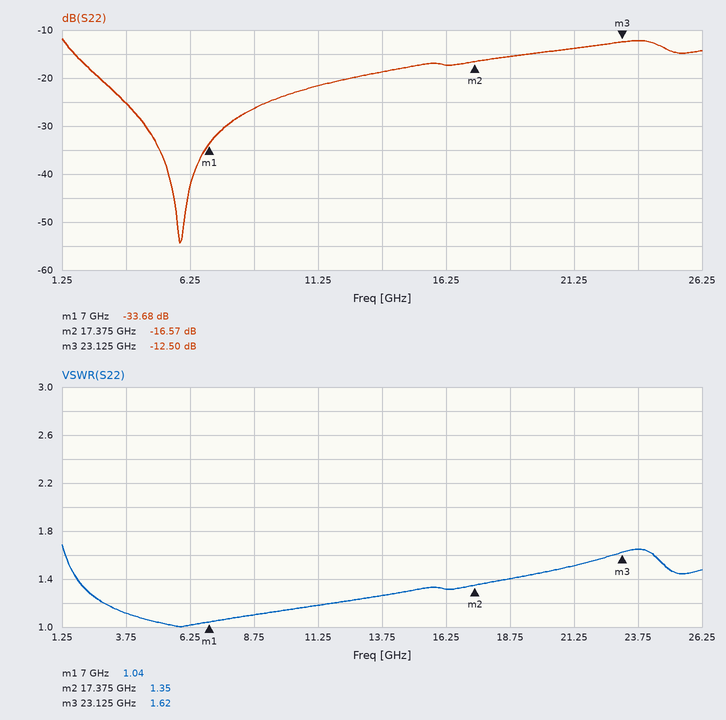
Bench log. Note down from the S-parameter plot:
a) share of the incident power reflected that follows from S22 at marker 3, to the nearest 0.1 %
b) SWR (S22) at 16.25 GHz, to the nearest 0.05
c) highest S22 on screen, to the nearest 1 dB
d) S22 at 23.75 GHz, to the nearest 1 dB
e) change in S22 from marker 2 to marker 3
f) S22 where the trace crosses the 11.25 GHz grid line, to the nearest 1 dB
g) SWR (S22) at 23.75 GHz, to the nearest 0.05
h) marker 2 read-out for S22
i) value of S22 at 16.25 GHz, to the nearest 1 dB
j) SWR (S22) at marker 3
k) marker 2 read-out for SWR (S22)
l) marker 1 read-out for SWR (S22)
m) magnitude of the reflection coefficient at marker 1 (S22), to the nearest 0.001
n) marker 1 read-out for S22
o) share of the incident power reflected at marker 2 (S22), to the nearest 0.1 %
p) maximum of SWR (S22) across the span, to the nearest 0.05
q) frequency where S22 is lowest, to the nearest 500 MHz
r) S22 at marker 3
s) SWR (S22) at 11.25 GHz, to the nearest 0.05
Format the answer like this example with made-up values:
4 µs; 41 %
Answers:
5.6 %; 1.30; -12 dB; -12 dB; 4.07 dB; -22 dB; 1.65; -16.57 dB; -17 dB; 1.62; 1.35; 1.04; 0.021; -33.68 dB; 2.2 %; 1.70; 6.0 GHz; -12.50 dB; 1.20
